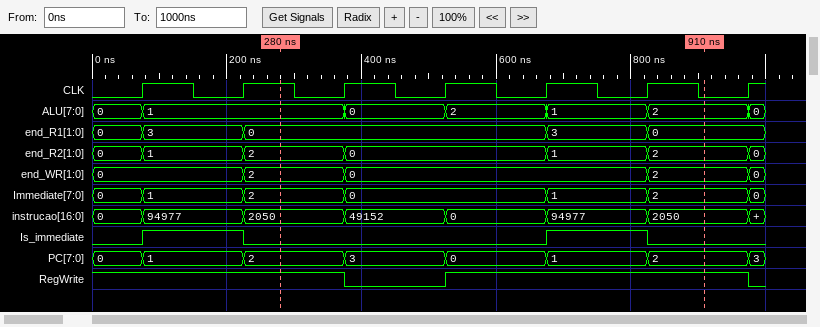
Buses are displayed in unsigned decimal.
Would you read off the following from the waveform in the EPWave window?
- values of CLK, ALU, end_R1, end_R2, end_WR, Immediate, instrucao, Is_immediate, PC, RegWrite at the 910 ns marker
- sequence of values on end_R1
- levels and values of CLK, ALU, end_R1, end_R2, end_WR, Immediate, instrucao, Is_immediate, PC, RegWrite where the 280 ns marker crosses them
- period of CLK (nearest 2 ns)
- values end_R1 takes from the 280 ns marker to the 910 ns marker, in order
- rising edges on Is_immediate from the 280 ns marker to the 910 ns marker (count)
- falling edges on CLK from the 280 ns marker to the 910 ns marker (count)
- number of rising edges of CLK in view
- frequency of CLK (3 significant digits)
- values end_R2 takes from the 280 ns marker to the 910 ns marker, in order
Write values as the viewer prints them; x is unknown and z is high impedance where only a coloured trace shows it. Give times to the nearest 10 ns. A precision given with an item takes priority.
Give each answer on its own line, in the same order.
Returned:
CLK=0, ALU=2, end_R1=0, end_R2=2, end_WR=2, Immediate=2, instrucao=2050, Is_immediate=0, PC=2, RegWrite=1
0, 3, 0, 3, 0
CLK=1, ALU=1, end_R1=0, end_R2=2, end_WR=2, Immediate=2, instrucao=2050, Is_immediate=0, PC=2, RegWrite=1
150 ns
0, 3, 0
1
5
7
6.67 MHz
2, 0, 1, 2
